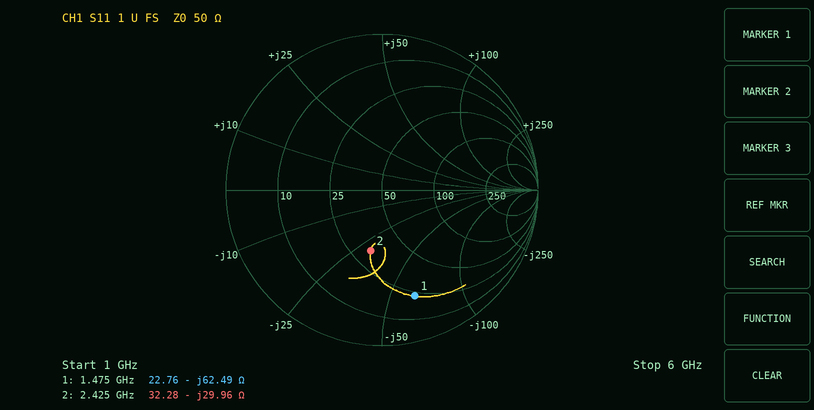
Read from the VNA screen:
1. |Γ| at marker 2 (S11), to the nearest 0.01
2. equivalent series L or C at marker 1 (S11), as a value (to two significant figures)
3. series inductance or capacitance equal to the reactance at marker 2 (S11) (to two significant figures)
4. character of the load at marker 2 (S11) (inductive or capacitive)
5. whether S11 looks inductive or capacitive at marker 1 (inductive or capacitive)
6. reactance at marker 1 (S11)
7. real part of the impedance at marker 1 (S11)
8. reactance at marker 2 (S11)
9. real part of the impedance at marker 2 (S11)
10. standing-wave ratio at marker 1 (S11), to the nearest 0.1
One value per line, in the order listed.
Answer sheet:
0.40
1.7 pF
2.2 pF
capacitive
capacitive
-62.49 Ω
22.76 Ω
-29.96 Ω
32.28 Ω
5.9
